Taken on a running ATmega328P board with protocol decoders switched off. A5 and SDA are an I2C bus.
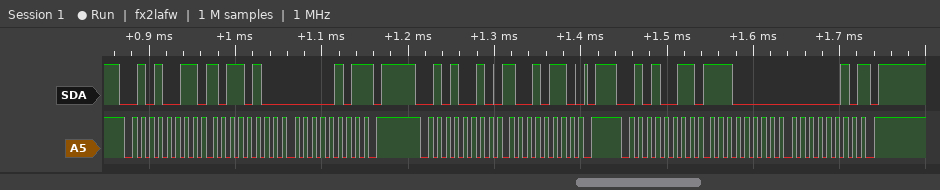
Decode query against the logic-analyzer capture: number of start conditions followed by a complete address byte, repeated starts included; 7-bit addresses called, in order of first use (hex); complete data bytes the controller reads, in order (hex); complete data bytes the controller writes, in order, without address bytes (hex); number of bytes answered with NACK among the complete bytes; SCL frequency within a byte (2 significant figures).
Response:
3
0x29
B4 05 E0 02
96
2
100 kHz
